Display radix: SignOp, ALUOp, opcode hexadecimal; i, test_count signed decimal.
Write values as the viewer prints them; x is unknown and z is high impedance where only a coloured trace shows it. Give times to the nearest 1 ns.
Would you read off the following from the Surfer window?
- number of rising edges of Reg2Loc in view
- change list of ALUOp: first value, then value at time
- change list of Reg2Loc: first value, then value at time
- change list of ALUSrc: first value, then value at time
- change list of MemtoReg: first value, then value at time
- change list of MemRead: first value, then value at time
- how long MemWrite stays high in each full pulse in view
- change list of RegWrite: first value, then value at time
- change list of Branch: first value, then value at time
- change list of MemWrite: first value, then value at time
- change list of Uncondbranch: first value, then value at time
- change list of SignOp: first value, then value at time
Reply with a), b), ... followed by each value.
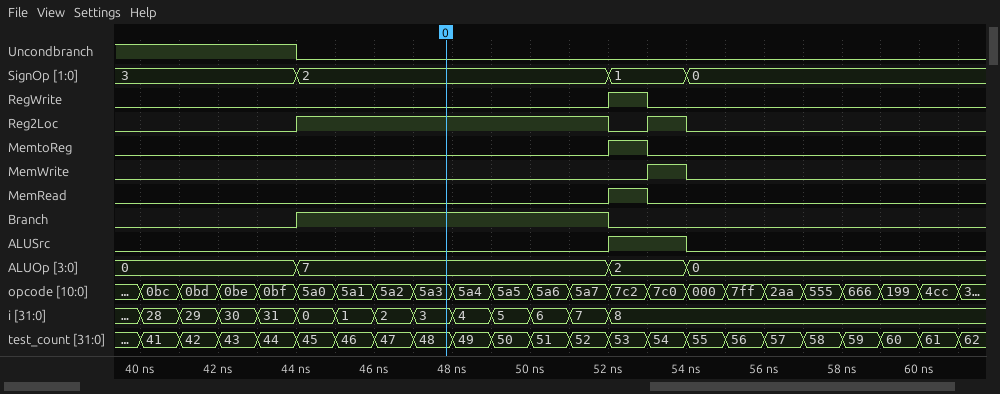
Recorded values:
a) 2
b) 0, 7 at 44 ns, 2 at 52 ns, 0 at 54 ns
c) 0, 1 at 44 ns, 0 at 52 ns, 1 at 53 ns, 0 at 54 ns
d) 0, 1 at 52 ns, 0 at 54 ns
e) 0, 1 at 52 ns, 0 at 53 ns
f) 0, 1 at 52 ns, 0 at 53 ns
g) 1 ns
h) 0, 1 at 52 ns, 0 at 53 ns
i) 0, 1 at 44 ns, 0 at 52 ns
j) 0, 1 at 53 ns, 0 at 54 ns
k) 1, 0 at 44 ns
l) 3, 2 at 44 ns, 1 at 52 ns, 0 at 54 ns
